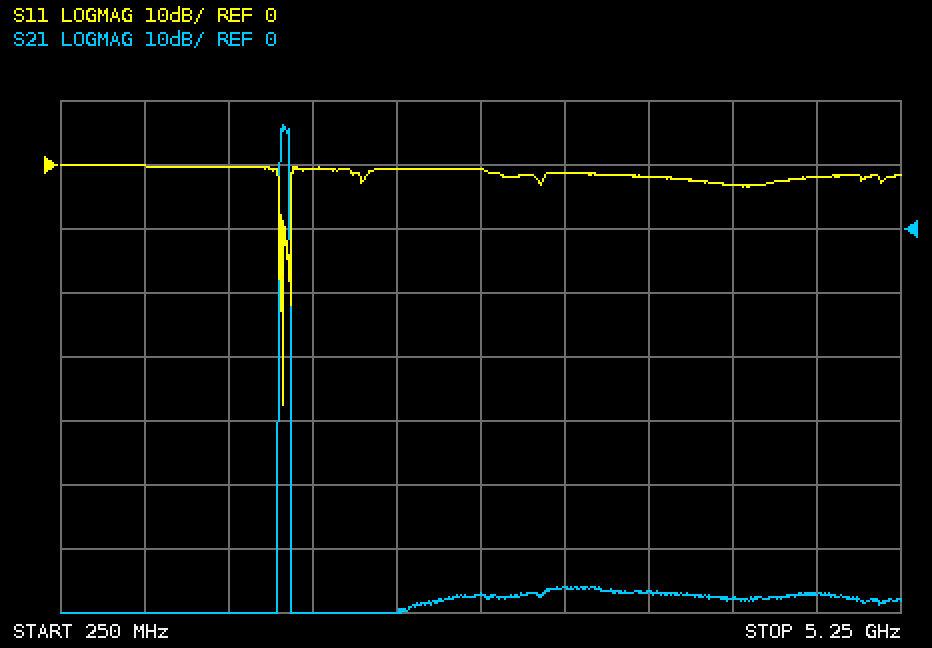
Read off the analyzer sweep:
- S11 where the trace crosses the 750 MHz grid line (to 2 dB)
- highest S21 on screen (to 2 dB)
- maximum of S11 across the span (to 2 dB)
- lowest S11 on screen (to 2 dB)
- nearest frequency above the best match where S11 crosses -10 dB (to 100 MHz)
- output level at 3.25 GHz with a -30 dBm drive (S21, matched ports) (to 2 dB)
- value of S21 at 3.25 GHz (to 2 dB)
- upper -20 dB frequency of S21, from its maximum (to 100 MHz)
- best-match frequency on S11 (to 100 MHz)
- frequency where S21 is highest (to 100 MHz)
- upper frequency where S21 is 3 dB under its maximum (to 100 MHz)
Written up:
0 dB
16 dB
0 dB
-38 dB
1.6 GHz
-86 dBm
-56 dB
1.6 GHz
1.6 GHz
1.6 GHz
1.6 GHz
